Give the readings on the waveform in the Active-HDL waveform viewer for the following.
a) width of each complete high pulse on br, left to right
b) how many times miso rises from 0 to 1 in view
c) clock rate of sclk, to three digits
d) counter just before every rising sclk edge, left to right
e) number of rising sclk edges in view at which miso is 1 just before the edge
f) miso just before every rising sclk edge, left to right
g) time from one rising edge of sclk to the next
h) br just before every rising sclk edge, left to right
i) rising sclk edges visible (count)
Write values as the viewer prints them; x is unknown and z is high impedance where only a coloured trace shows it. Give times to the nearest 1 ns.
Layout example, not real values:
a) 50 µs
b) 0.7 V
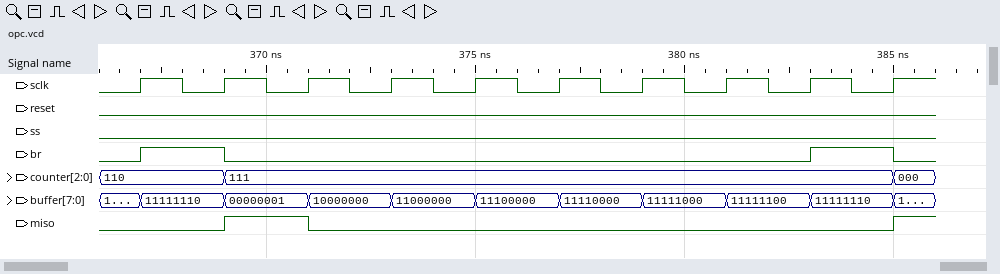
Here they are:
a) 2 ns, 2 ns
b) 2
c) 500 MHz
d) 110, 110, 111, 111, 111, 111, 111, 111, 111, 111
e) 1
f) 0 0 1 0 0 0 0 0 0 0
g) 2 ns
h) 0 1 0 0 0 0 0 0 0 1
i) 10
